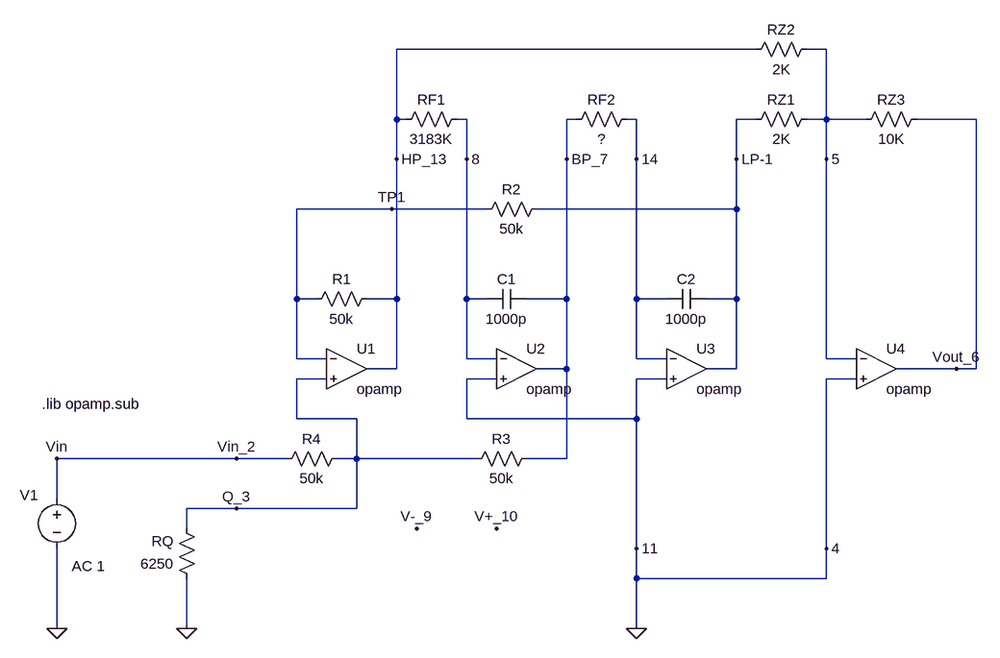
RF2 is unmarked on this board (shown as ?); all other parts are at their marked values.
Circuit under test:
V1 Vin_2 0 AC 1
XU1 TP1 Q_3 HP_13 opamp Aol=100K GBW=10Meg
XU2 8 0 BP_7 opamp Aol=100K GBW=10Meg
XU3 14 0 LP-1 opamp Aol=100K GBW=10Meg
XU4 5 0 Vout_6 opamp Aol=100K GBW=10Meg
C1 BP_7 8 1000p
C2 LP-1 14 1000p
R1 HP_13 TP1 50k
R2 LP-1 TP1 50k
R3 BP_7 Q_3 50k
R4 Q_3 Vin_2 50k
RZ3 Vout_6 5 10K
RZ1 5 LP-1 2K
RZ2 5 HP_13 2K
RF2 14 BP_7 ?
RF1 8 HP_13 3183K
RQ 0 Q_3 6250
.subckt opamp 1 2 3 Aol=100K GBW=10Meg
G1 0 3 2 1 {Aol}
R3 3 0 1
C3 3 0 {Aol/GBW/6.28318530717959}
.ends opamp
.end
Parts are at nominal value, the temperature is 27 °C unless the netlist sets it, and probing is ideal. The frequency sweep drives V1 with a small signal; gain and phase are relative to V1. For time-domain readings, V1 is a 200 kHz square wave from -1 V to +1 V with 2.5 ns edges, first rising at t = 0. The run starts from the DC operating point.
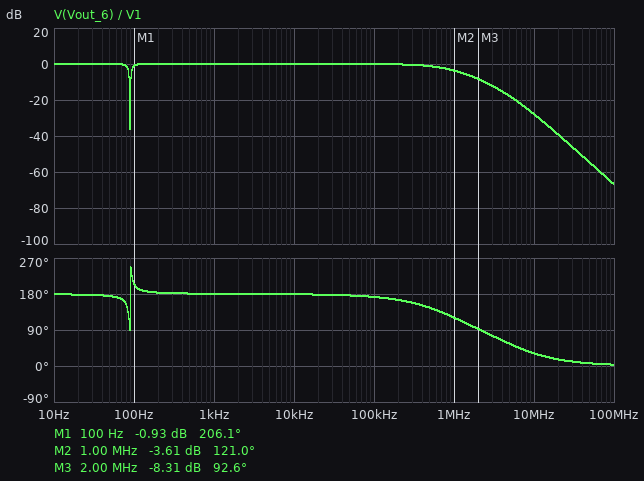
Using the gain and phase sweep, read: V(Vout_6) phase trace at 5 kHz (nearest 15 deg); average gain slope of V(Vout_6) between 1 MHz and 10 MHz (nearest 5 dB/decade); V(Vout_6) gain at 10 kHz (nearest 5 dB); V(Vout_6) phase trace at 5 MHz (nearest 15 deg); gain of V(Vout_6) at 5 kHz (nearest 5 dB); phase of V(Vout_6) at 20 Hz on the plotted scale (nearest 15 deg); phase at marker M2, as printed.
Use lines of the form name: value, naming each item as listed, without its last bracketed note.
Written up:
V(Vout_6) phase trace at 5 kHz: 180 deg
average gain slope of V(Vout_6) between 1 MHz and 10 MHz: -25 dB/decade
V(Vout_6) gain at 10 kHz: 0 dB
V(Vout_6) phase trace at 5 MHz: 60 deg
gain of V(Vout_6) at 5 kHz: 0 dB
phase of V(Vout_6) at 20 Hz on the plotted scale: 180 deg
phase at marker M2, as printed: 121.0 deg
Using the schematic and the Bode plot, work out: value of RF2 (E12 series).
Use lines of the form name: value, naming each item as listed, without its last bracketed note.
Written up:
value of RF2: 1 MΩ
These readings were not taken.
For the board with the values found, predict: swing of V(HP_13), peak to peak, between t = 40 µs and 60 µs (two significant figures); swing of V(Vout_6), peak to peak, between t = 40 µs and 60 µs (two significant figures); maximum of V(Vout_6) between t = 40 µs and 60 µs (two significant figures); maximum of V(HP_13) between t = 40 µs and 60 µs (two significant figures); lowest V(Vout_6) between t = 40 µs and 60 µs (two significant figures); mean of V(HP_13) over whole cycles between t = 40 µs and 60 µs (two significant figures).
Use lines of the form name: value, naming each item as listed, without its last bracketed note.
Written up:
swing of V(HP_13), peak to peak, between t = 40 µs and 60 µs: 400 mV
swing of V(Vout_6), peak to peak, between t = 40 µs and 60 µs: 2.0 V
maximum of V(Vout_6) between t = 40 µs and 60 µs: 1.0 V
maximum of V(HP_13) between t = 40 µs and 60 µs: 400 mV
lowest V(Vout_6) between t = 40 µs and 60 µs: -1.0 V
mean of V(HP_13) over whole cycles between t = 40 µs and 60 µs: 200 mV
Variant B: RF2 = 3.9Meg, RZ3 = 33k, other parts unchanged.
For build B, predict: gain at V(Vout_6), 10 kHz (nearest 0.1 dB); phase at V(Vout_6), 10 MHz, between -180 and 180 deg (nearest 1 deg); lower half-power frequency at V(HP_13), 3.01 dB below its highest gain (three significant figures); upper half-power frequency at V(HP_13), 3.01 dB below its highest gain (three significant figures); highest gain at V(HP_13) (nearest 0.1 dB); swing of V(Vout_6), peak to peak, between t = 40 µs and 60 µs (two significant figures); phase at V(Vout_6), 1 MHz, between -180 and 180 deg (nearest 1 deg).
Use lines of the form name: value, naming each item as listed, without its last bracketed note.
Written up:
gain at V(Vout_6), 10 kHz: 10.4 dB
phase at V(Vout_6), 10 MHz, between -180 and 180 deg: 28 deg
lower half-power frequency at V(HP_13), 3.01 dB below its highest gain: 41.3 Hz
upper half-power frequency at V(HP_13), 3.01 dB below its highest gain: 52.0 Hz
highest gain at V(HP_13): -0.8 dB
swing of V(Vout_6), peak to peak, between t = 40 µs and 60 µs: 6.5 V
phase at V(Vout_6), 1 MHz, between -180 and 180 deg: 95 deg
